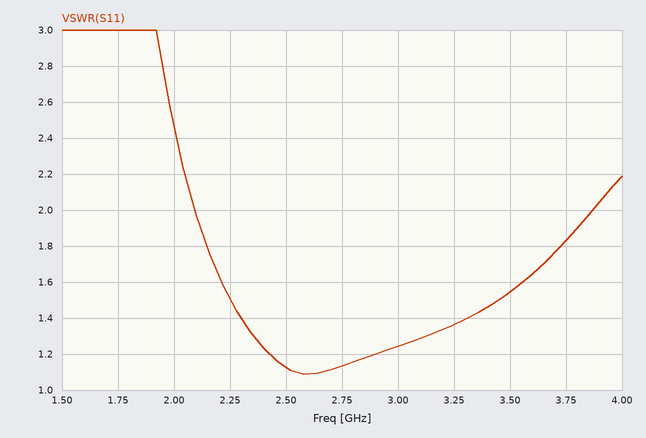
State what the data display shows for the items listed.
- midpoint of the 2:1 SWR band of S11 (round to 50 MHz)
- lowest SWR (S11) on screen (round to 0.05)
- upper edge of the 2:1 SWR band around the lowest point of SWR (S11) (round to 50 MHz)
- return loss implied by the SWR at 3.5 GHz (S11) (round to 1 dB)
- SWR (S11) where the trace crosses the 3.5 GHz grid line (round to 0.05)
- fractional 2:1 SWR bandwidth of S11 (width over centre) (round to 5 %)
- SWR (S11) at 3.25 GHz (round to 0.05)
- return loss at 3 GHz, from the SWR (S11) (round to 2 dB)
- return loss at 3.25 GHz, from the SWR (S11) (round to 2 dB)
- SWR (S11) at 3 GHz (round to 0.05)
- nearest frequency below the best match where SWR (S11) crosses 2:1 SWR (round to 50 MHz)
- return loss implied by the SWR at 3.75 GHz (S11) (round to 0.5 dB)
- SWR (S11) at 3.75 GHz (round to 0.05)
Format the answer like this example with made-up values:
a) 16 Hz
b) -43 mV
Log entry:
a) 3.00 GHz
b) 1.10
c) 3.85 GHz
d) 13 dB
e) 1.55
f) 60 %
g) 1.35
h) 20 dB
i) 16 dB
j) 1.25
k) 2.10 GHz
l) 10.5 dB
m) 1.85
